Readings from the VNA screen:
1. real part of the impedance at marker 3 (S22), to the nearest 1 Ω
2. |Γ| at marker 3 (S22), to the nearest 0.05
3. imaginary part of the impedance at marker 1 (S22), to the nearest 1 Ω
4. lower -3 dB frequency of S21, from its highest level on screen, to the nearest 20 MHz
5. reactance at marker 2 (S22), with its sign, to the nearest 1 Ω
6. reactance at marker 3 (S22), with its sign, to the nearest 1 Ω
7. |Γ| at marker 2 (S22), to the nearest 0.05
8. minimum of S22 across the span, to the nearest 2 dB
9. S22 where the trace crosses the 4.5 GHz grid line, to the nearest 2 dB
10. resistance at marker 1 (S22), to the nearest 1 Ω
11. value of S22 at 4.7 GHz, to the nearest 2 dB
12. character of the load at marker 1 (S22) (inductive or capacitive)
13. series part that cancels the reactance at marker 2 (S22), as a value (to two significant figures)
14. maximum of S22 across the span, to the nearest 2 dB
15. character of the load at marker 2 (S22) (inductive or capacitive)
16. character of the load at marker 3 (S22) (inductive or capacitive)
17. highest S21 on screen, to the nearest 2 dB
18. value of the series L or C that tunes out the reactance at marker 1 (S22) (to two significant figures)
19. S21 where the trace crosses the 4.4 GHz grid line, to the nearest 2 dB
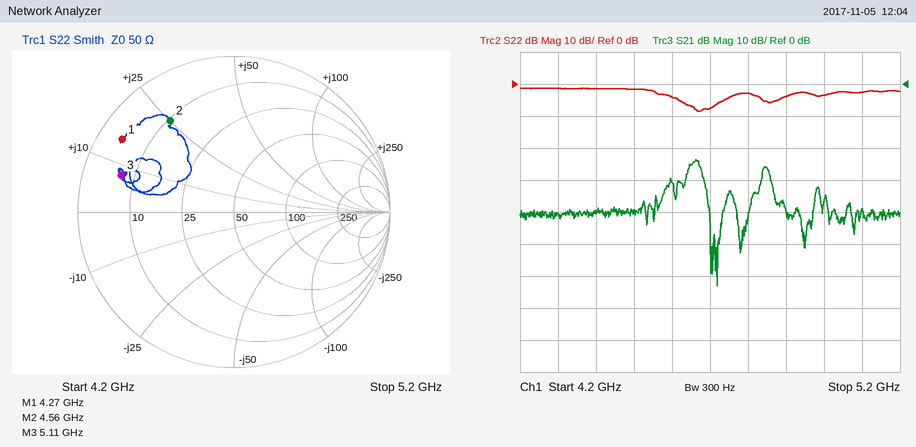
7 Ω
0.75
+15 Ω
4.64 GHz
+25 Ω
+8 Ω
0.70
-8 dB
-2 dB
4 Ω
-8 dB
inductive
1.4 pF
-2 dB
inductive
inductive
-24 dB
2.5 pF
-40 dB
